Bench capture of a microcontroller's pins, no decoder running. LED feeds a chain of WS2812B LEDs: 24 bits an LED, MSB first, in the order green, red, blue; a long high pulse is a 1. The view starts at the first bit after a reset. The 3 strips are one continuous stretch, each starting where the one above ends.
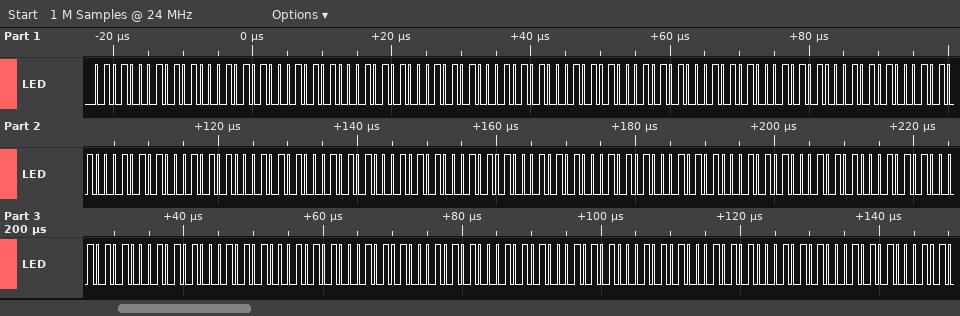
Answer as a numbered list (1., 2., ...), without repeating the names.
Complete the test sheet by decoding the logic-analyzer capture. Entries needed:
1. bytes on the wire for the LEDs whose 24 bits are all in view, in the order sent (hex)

1. 51 51 51 51 51 51 51 51 51 51 51 51 51 51 51 51 51 51 51 51 51 51 51 51 51 51 51 51 51 51 51 51 51 51 51 51
